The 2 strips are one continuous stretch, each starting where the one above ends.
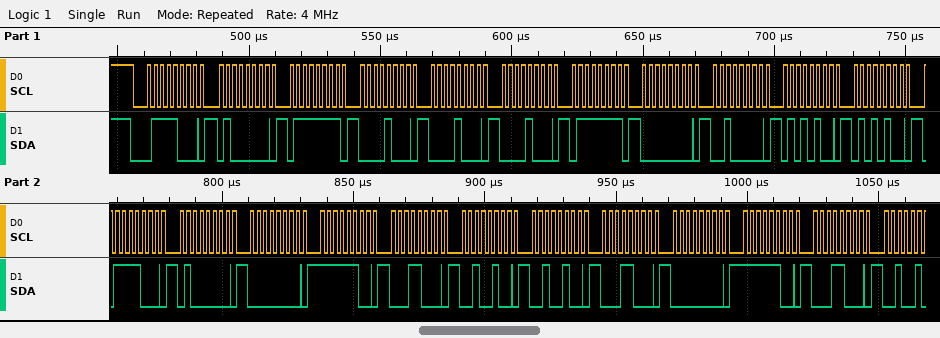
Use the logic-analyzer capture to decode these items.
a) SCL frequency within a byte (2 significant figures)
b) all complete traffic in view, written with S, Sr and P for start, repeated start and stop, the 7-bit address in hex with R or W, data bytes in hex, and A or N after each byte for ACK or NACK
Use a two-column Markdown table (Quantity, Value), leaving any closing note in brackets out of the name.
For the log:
| Quantity | Value |
|---|---|
| SCL frequency within a byte | 400 kHz |
| all complete traffic in view, written with S, Sr and P for start, repeated start and stop, the 7-bit address in hex with R or W, data bytes in hex, and A or N after each byte for ACK or NACK | S 3CW A 40 A 7F A 08 A 08 A 08 A 7F A 00 A 20 A 54 A 54 A 78 A 40 A 00 A FC A 18 A 24 A 24 A 18 A 00 A FC A 18 A |
